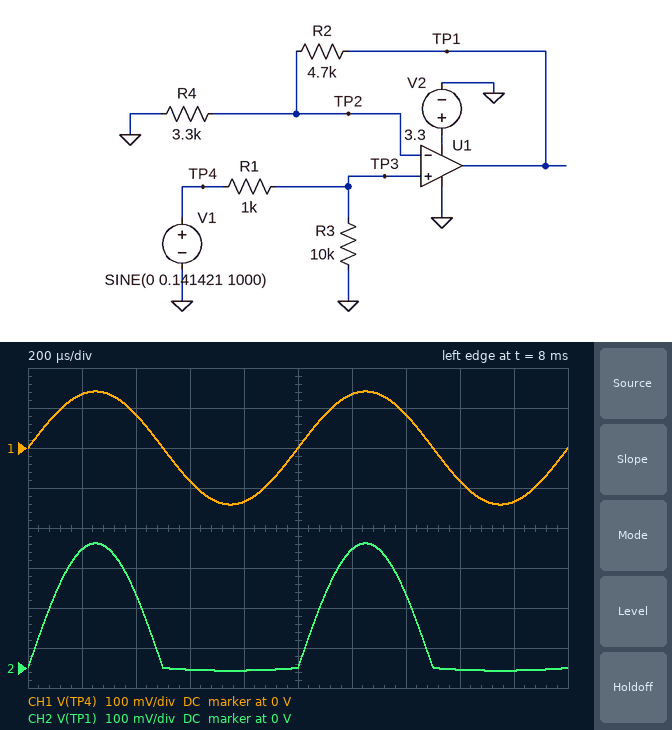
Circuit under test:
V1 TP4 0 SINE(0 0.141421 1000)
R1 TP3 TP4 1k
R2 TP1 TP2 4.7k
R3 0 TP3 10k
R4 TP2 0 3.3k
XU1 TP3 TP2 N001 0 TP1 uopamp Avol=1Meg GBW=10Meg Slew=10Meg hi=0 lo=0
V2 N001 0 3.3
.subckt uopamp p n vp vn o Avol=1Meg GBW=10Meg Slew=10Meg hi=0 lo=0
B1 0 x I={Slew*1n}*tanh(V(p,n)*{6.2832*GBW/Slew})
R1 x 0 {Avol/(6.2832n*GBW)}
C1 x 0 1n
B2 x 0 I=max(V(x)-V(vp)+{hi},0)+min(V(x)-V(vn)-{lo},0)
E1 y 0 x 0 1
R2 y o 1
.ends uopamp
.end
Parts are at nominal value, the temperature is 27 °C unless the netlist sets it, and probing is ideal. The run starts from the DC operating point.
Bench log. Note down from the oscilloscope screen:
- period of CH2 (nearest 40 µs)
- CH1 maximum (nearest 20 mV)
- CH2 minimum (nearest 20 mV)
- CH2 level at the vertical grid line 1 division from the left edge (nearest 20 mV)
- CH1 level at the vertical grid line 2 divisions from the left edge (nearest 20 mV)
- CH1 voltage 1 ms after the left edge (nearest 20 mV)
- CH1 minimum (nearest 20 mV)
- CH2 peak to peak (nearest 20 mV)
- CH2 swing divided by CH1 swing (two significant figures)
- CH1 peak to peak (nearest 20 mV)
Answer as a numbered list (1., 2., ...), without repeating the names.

1. 1.00 ms
2. 140 mV
3. 0 V
4. 300 mV
5. 80 mV
6. 0 V
7. -140 mV
8. 320 mV
9. 1.1
10. 280 mV
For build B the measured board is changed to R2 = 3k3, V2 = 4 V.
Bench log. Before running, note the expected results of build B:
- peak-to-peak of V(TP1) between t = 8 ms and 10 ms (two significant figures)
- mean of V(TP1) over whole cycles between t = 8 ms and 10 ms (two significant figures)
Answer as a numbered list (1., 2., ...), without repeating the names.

1. 260 mV
2. 80 mV
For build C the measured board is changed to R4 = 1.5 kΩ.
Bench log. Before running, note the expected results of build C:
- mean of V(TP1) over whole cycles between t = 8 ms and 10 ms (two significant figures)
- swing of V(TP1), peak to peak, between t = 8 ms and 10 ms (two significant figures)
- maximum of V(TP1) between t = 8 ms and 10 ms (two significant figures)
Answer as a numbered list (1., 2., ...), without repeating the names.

1. 170 mV
2. 540 mV
3. 530 mV
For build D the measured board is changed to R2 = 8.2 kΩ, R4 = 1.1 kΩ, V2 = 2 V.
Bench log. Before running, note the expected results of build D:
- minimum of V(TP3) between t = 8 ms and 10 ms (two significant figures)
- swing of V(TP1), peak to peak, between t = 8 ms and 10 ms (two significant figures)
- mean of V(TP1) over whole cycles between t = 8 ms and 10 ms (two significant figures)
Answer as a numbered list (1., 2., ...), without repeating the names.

1. -130 mV
2. 1.1 V
3. 340 mV
